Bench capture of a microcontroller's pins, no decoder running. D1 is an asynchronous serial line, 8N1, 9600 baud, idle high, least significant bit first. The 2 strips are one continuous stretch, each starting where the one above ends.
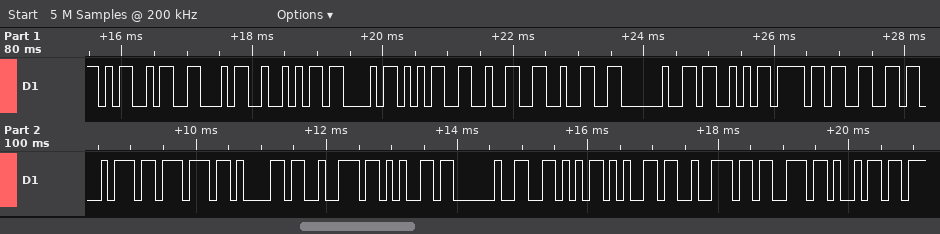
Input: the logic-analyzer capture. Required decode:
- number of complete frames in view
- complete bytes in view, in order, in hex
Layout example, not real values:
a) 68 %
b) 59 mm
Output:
a) 22
b) 4D 46 52 43 35 32 32 20 53 6F 66 74 77 61 72 65 20 56 65 72 73 69
